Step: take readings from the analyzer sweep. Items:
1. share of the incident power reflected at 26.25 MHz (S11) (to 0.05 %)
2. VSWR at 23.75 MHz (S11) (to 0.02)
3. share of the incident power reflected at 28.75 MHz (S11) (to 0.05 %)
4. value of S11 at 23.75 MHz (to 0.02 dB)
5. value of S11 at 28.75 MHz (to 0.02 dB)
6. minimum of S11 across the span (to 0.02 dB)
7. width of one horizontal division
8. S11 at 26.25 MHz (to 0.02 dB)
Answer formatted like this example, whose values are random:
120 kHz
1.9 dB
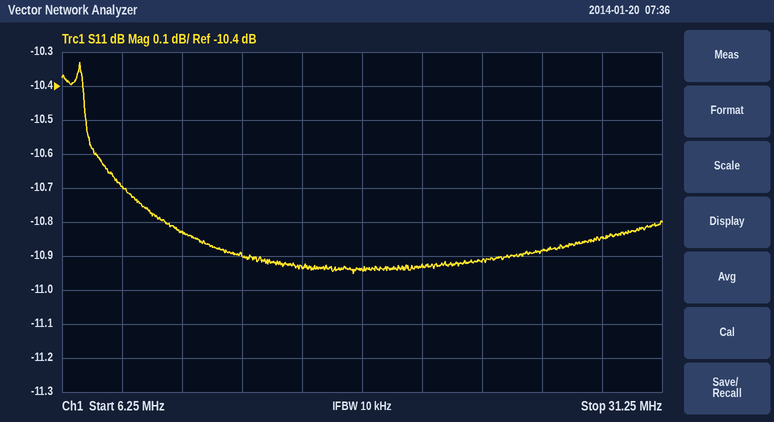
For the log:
8.15 %
1.80
8.25 %
-10.92 dB
-10.84 dB
-10.96 dB
2.5 MHz
-10.88 dB
